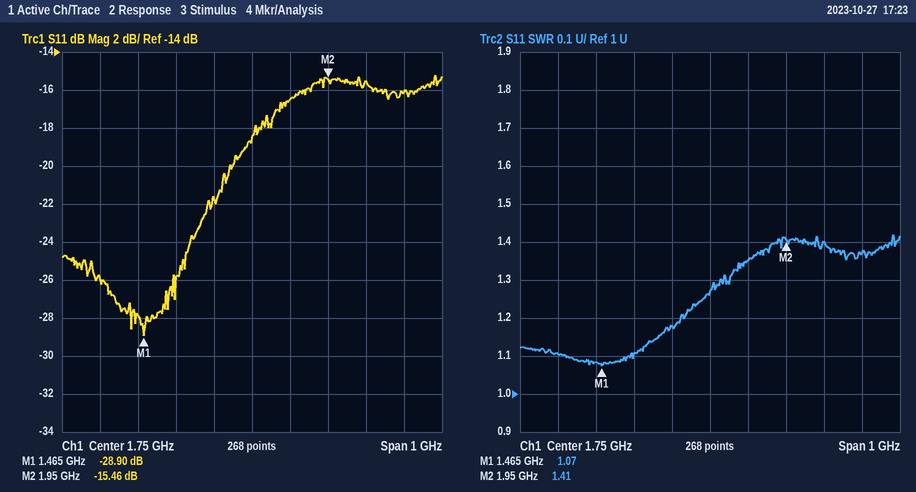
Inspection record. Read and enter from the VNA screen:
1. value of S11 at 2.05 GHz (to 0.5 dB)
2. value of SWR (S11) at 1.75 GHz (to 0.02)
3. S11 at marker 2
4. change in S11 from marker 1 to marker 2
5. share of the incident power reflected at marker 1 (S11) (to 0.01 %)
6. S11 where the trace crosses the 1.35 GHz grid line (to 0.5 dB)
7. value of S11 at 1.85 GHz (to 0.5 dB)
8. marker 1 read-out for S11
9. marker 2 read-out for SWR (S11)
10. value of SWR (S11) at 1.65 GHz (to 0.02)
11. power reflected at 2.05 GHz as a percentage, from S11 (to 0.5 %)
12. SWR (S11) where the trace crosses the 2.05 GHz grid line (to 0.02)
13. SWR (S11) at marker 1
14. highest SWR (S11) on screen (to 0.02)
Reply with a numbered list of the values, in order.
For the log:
1. -15.5 dB
2. 1.26
3. -15.46 dB
4. 13.44 dB
5. 0.13 %
6. -26.0 dB
7. -16.5 dB
8. -28.90 dB
9. 1.41
10. 1.18
11. 3.0 %
12. 1.40
13. 1.07
14. 1.42
